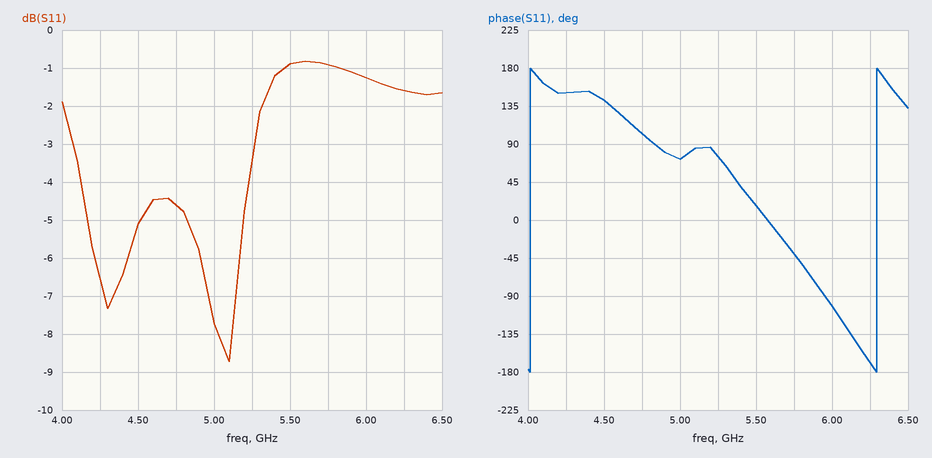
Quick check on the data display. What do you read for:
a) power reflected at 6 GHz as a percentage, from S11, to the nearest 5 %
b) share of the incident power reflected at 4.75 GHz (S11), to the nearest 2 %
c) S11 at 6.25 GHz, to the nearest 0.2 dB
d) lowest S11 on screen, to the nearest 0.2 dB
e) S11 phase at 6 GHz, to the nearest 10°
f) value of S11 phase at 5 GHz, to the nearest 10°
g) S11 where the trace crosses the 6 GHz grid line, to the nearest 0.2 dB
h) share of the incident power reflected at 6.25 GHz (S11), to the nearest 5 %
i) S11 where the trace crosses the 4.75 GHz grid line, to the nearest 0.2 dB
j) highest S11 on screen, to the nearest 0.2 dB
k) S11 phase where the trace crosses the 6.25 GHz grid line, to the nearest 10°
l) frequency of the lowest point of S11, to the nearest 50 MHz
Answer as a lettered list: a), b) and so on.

a) 75 %
b) 34 %
c) -1.6 dB
d) -8.8 dB
e) -100°
f) 70°
g) -1.2 dB
h) 70 %
i) -4.6 dB
j) -0.8 dB
k) -170°
l) 5.10 GHz
